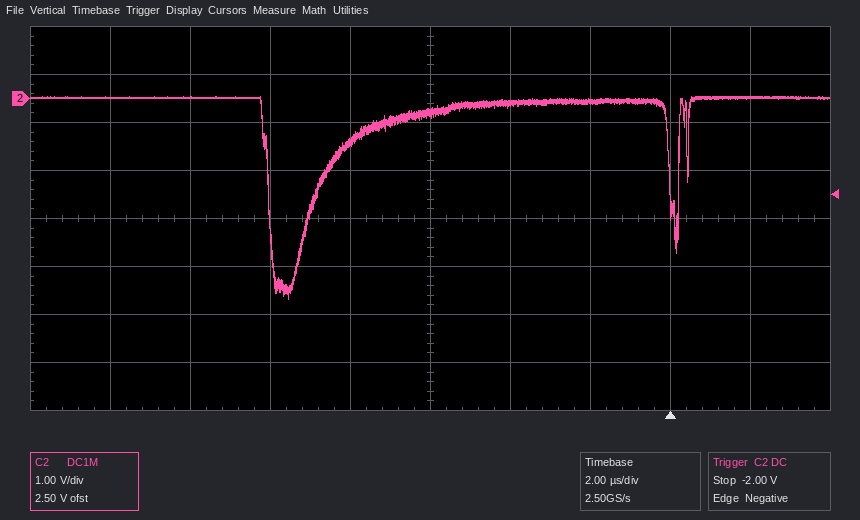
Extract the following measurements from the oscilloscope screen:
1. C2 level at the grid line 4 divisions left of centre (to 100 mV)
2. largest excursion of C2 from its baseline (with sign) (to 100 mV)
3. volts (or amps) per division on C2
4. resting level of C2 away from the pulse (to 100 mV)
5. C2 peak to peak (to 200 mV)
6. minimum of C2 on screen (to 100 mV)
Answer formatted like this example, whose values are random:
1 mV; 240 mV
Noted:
0.0 V; -4.2 V; 1 V; 0.0 V; 4.2 V; -4.2 V
